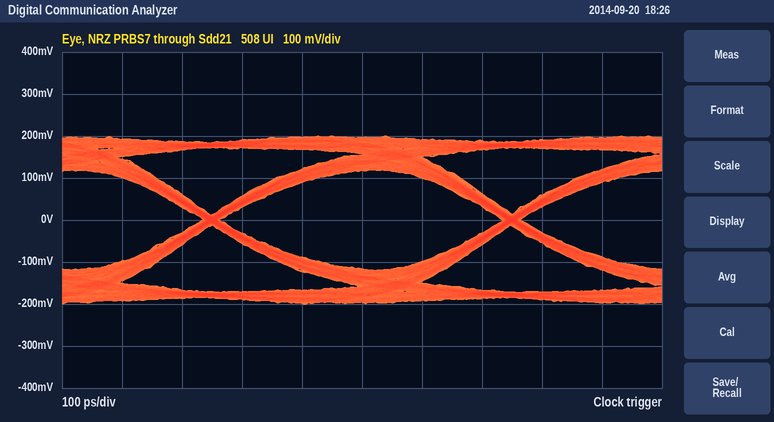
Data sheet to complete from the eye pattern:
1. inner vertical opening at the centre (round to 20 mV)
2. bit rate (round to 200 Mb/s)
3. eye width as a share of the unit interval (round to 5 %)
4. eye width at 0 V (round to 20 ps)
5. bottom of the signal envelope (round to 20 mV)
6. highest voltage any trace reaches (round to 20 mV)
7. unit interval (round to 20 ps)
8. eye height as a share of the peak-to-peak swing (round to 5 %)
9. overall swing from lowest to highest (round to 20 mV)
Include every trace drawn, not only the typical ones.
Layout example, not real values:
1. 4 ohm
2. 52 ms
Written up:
1. 240 mV
2. 2.0 Gb/s
3. 95 %
4. 480 ps
5. -200 mV
6. 200 mV
7. 500 ps
8. 60 %
9. 400 mV
